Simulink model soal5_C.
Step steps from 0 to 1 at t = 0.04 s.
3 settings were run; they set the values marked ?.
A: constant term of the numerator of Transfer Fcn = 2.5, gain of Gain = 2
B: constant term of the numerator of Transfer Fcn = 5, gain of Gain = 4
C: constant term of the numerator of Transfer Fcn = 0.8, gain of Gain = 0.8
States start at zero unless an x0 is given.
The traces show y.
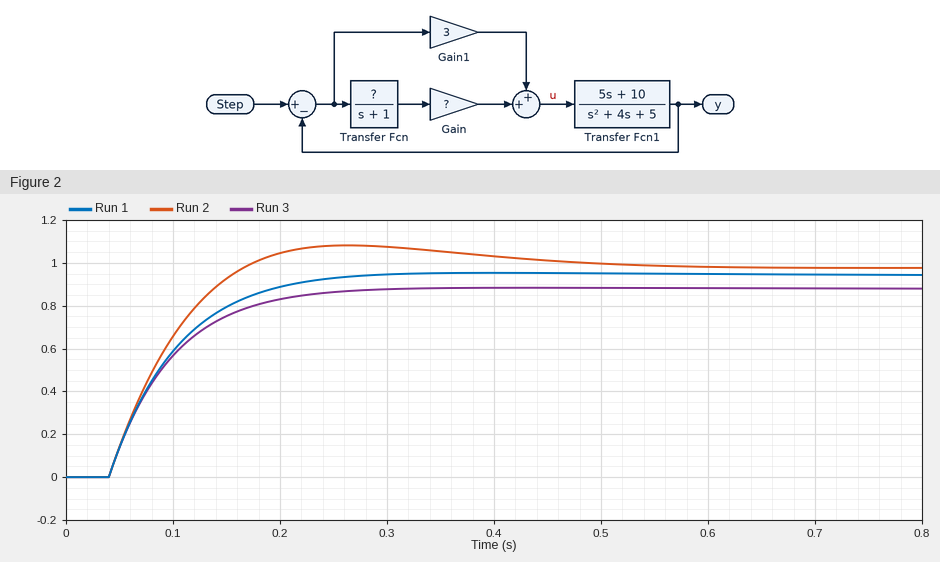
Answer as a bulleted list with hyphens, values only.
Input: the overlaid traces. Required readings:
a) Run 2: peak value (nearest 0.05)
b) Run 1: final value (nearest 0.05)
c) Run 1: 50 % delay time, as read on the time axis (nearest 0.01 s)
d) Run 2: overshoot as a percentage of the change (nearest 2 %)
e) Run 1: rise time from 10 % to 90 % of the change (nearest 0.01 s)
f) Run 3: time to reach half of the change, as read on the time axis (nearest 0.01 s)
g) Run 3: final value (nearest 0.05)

- 1.10
- 0.95
- 0.08 s
- 10 %
- 0.13 s
- 0.08 s
- 0.90
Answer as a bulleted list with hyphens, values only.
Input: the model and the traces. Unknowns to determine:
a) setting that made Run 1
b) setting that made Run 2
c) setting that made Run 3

- A
- B
- C
